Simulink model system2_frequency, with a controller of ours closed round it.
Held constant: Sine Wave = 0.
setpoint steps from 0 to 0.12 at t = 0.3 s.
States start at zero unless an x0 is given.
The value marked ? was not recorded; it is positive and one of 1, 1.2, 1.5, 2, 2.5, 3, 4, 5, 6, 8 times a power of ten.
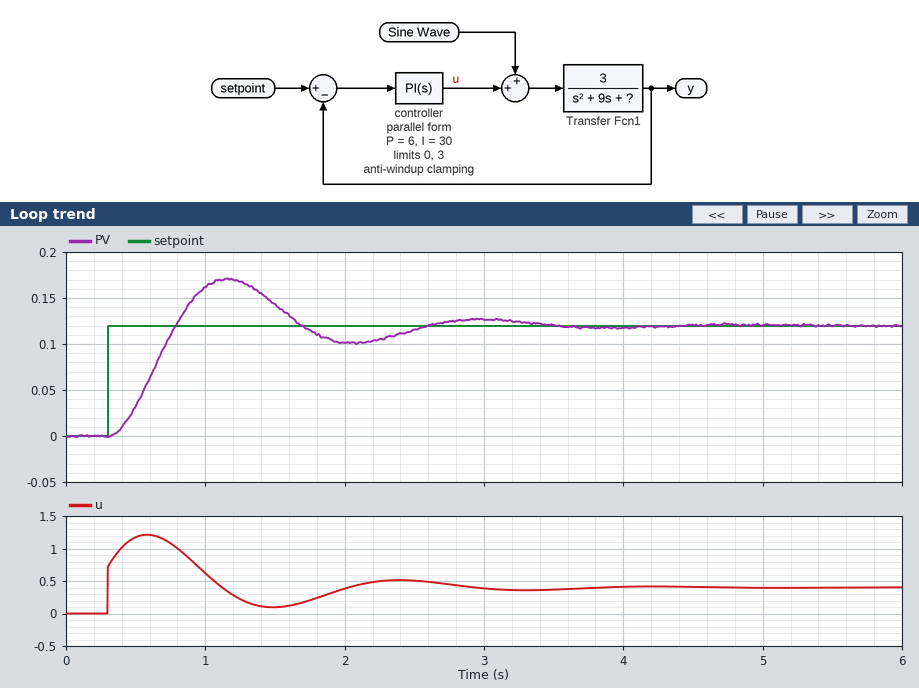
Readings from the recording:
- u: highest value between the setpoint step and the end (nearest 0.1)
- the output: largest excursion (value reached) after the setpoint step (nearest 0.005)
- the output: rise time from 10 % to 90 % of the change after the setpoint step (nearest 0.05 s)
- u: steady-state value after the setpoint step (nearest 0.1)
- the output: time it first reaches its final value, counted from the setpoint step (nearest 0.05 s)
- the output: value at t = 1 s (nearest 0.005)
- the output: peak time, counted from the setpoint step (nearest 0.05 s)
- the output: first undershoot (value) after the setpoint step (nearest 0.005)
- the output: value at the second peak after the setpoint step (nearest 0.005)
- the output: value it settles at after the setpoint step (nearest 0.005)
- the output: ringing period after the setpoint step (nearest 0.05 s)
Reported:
1.2
0.170
0.35 s
0.4
0.50 s
0.160
0.85 s
0.100
0.125
0.120
1.80 s
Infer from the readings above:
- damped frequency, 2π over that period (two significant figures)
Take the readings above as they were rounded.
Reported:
3.5 rad/s
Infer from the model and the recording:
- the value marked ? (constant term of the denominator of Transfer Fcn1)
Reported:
10
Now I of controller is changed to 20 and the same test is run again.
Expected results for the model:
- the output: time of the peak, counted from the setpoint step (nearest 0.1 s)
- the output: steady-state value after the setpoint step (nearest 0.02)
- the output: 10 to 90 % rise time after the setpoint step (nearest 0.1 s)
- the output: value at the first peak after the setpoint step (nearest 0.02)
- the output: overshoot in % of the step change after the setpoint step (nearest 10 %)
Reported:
1.0 s
0.12
0.4 s
0.16
30 %
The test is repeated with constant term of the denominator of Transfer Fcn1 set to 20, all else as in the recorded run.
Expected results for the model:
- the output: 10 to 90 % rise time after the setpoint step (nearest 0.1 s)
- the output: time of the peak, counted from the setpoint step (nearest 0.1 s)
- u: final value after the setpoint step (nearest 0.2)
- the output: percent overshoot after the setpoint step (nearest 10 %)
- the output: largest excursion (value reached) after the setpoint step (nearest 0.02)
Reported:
0.4 s
0.8 s
0.8
20 %
0.14
